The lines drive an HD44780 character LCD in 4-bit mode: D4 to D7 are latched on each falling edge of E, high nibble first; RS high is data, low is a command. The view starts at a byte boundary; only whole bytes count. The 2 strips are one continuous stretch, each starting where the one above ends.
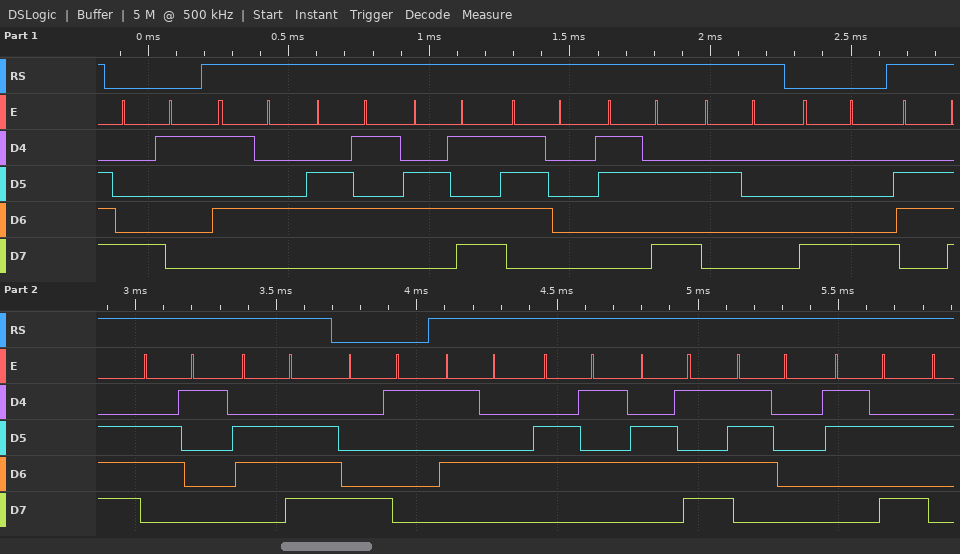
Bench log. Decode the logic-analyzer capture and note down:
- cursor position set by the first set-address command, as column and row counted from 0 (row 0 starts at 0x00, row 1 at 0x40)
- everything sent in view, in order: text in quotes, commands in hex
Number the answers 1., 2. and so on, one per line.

1. column 1, row 0
2. 0x81 "Temp: " 0x88 "nan" 0x81 "Temp:"
